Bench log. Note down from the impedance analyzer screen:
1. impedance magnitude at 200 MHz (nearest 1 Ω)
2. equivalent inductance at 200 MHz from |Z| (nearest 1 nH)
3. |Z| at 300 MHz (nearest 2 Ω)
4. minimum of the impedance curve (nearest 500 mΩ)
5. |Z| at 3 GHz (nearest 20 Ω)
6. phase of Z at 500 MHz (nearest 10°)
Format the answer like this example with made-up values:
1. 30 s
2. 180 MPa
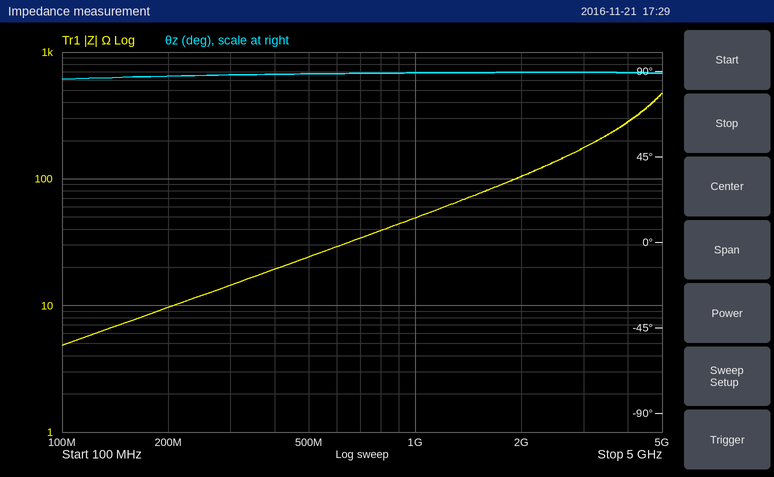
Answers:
1. 10 Ω
2. 8 nH
3. 14 Ω
4. 5.0 Ω
5. 180 Ω
6. 90°
